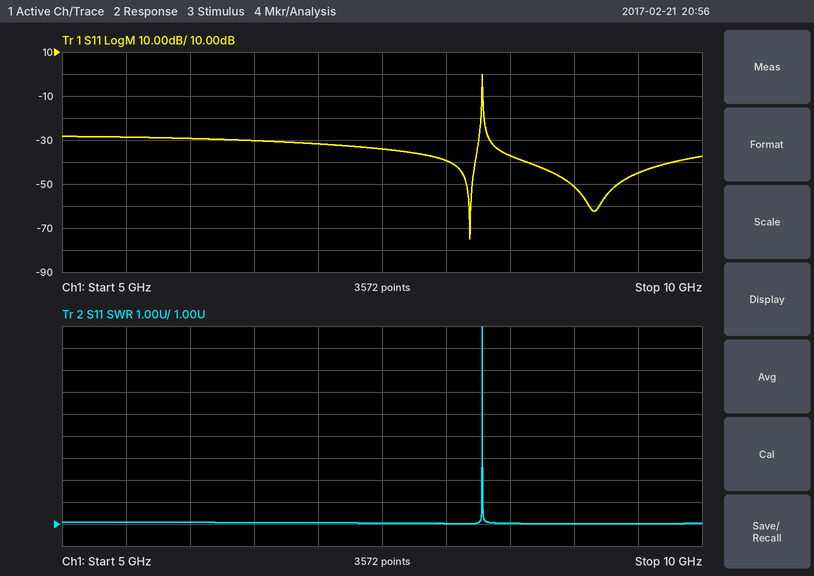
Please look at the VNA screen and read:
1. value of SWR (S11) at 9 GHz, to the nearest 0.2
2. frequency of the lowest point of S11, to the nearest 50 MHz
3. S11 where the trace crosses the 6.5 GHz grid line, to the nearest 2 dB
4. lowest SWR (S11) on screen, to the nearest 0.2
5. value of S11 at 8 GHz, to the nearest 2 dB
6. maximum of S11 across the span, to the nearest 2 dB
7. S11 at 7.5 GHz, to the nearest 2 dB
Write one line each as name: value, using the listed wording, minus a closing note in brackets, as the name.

value of SWR (S11) at 9 GHz, to the nearest 0.2: 1.0
frequency of the lowest point of S11, to the nearest 50 MHz: 8.20 GHz
S11 where the trace crosses the 6.5 GHz grid line, to the nearest 2 dB: -30 dB
lowest SWR (S11) on screen, to the nearest 0.2: 1.0
value of S11 at 8 GHz, to the nearest 2 dB: -40 dB
maximum of S11 across the span, to the nearest 2 dB: 0 dB
S11 at 7.5 GHz, to the nearest 2 dB: -34 dB
